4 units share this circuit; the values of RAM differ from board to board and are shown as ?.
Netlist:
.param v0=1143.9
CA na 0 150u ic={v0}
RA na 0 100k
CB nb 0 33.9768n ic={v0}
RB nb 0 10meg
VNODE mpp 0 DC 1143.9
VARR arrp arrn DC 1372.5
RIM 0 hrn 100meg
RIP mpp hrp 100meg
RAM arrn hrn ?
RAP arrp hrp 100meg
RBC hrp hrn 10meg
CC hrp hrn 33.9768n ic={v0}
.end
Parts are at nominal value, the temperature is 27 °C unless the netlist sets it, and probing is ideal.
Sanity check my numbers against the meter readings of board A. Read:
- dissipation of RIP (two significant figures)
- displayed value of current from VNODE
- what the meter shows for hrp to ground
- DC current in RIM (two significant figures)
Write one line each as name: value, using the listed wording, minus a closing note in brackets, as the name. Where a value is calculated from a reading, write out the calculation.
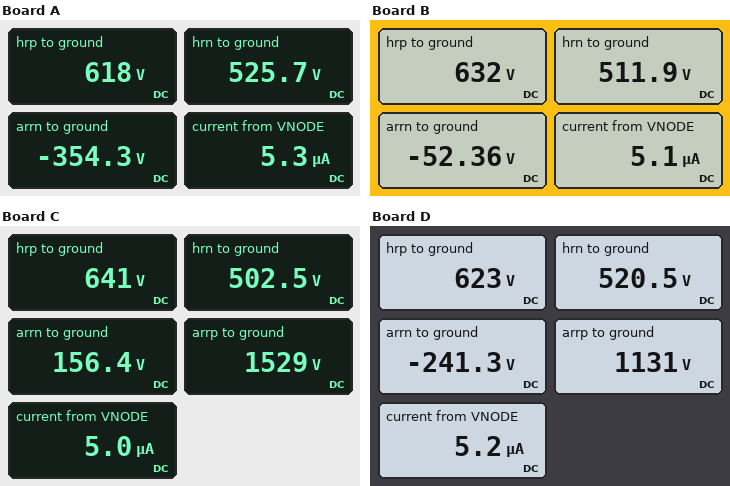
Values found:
dissipation of RIP: (1.144 kV - 618 V)^2 / 100 MΩ = 2.8 mW
displayed value of current from VNODE: 5.3 µA
what the meter shows for hrp to ground: 618 V
DC current in RIM: (525.7 V) / 100 MΩ = 5.3 µA
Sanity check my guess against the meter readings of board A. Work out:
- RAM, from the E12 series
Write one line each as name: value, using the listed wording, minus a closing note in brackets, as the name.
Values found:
RAM, from the E12 series: 220 MΩ
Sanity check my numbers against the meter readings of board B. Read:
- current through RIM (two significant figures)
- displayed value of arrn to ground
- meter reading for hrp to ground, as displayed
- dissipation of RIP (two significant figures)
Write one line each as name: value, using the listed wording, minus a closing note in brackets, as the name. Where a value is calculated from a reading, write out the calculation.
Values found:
current through RIM: (511.9 V) / 100 MΩ = 5.1 µA
displayed value of arrn to ground: -52.36 V
meter reading for hrp to ground, as displayed: 632 V
dissipation of RIP: (1.144 kV - 632 V)^2 / 100 MΩ = 2.6 mW
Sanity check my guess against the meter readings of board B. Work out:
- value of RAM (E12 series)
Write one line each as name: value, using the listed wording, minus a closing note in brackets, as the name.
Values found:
value of RAM: 82 MΩ
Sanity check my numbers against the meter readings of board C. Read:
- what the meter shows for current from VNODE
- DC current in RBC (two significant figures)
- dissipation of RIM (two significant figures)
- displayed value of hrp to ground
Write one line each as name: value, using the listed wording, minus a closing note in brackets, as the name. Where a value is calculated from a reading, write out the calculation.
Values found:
what the meter shows for current from VNODE: 5.0 µA
DC current in RBC: (641 V - 502.5 V) / 10 MΩ = 14 µA
dissipation of RIM: (502.5 V)^2 / 100 MΩ = 2.5 mW
displayed value of hrp to ground: 641 V
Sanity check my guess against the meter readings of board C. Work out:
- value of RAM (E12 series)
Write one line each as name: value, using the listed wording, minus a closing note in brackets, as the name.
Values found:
value of RAM: 39 MΩ
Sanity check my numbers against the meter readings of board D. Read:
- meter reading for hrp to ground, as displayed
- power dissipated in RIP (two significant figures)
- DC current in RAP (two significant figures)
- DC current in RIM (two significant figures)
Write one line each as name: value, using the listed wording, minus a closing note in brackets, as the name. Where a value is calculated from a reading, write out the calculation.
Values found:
meter reading for hrp to ground, as displayed: 623 V
power dissipated in RIP: (1.144 kV - 623 V)^2 / 100 MΩ = 2.7 mW
DC current in RAP: (1.131 kV - 623 V) / 100 MΩ = 5.1 µA
DC current in RIM: (520.5 V) / 100 MΩ = 5.2 µA
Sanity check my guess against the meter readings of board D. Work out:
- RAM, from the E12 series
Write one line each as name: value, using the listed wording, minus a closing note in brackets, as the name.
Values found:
RAM, from the E12 series: 150 MΩ
